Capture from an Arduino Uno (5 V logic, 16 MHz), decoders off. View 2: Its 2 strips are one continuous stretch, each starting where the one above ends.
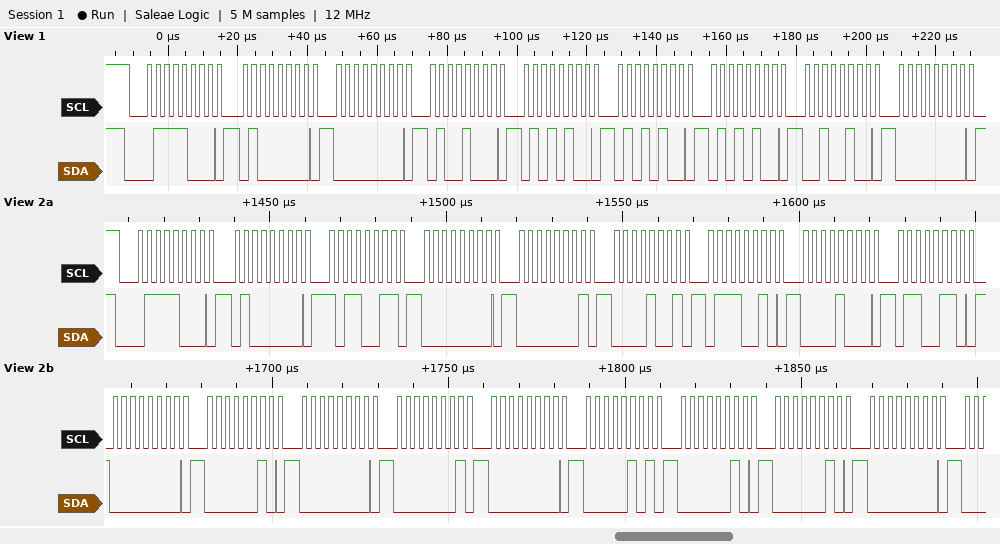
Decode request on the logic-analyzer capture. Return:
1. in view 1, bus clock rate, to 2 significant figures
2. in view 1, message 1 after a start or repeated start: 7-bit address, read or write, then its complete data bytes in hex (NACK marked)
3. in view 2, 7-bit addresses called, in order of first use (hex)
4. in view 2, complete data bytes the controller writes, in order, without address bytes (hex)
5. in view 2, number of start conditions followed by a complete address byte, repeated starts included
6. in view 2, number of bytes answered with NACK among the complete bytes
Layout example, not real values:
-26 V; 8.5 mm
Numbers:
400 kHz; 0x3C write: 40 00 48 54 54 54 24 00; 0x3C; 40 B3 00 01 09 72 08 66 00 02 00 01 00 05 02 02 00; 1; 0
